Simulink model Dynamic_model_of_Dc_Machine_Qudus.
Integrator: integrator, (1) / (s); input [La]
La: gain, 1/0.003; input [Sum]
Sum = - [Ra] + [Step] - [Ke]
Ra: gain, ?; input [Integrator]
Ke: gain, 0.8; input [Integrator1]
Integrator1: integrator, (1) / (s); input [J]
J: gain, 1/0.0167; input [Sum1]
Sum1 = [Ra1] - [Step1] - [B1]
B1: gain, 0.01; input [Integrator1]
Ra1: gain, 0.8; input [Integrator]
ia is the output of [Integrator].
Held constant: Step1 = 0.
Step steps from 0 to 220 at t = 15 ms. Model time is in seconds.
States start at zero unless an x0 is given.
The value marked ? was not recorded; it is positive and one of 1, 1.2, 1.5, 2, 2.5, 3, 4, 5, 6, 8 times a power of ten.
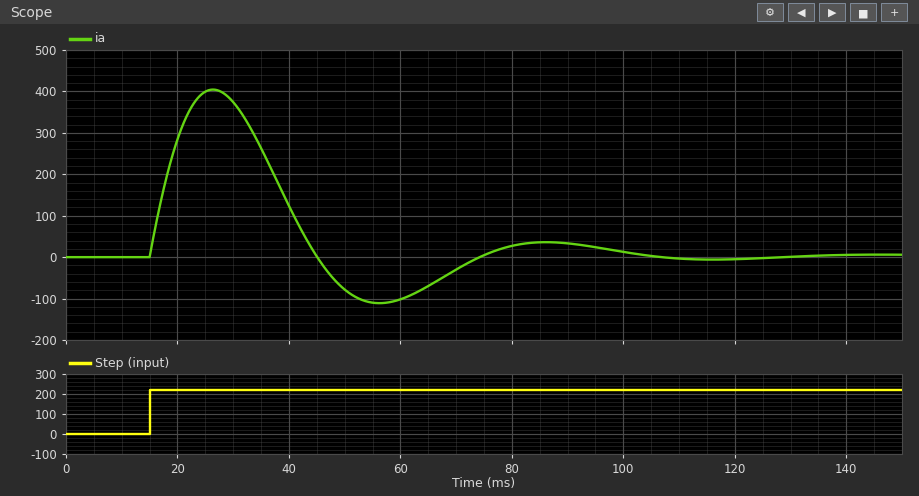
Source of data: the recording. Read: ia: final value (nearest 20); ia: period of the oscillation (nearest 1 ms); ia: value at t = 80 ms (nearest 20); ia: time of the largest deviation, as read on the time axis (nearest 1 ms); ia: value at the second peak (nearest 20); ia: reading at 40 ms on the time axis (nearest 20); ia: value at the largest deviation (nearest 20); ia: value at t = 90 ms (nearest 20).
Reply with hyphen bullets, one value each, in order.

- 0
- 60 ms
- 20
- 26 ms
- 40
- 120
- 400
- 40
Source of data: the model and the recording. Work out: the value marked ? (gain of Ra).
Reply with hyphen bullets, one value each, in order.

- 0.25
